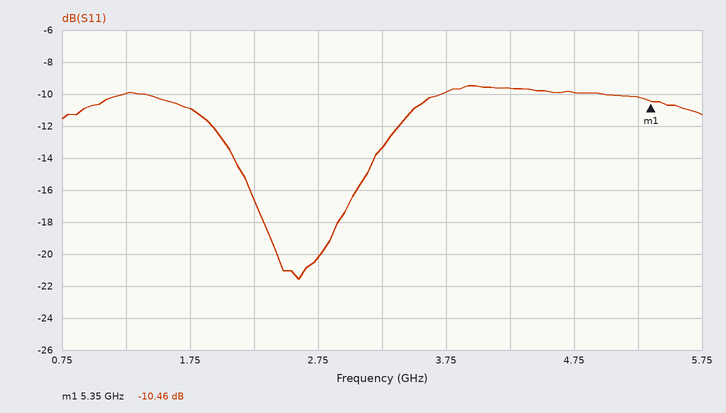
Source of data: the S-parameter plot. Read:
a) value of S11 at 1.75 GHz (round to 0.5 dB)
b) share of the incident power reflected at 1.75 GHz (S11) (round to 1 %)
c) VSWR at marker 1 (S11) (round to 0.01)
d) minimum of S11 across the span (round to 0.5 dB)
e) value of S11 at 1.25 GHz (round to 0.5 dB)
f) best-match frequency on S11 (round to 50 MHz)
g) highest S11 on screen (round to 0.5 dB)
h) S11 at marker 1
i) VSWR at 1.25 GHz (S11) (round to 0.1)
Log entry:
-11.0 dB
8 %
1.86
-21.5 dB
-10.0 dB
2.60 GHz
-9.5 dB
-10.46 dB
1.9
